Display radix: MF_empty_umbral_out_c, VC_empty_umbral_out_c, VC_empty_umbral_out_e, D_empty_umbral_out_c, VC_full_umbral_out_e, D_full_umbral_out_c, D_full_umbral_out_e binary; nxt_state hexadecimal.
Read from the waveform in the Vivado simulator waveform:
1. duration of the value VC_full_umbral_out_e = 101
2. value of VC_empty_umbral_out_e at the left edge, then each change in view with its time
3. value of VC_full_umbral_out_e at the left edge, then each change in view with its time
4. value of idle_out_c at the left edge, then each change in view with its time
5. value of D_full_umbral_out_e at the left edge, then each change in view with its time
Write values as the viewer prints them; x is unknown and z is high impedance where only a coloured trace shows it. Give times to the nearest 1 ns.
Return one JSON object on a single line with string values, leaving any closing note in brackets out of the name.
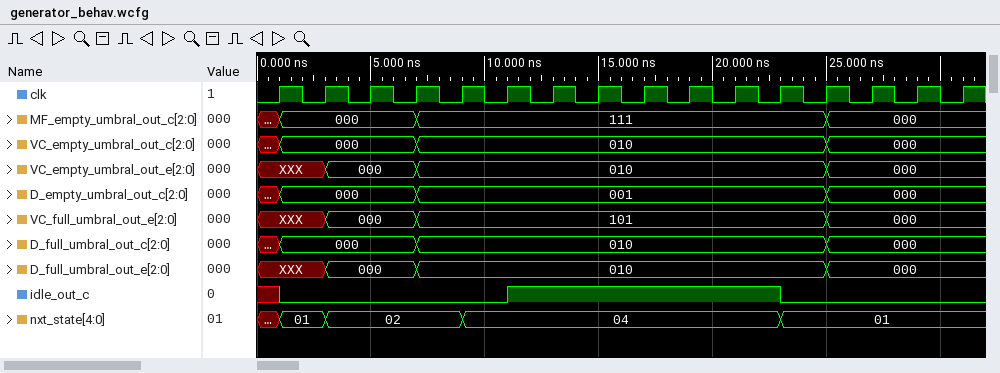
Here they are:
{"duration of the value VC_full_umbral_out_e = 101": "18 ns", "value of VC_empty_umbral_out_e at the left edge, then each change in view with its time": "XXX, 000 at 3 ns, 010 at 7 ns, 000 at 25 ns", "value of VC_full_umbral_out_e at the left edge, then each change in view with its time": "XXX, 000 at 3 ns, 101 at 7 ns, 000 at 25 ns", "value of idle_out_c at the left edge, then each change in view with its time": "x, 0 at 1 ns, 1 at 11 ns, 0 at 23 ns", "value of D_full_umbral_out_e at the left edge, then each change in view with its time": "XXX, 000 at 3 ns, 010 at 7 ns, 000 at 25 ns"}
